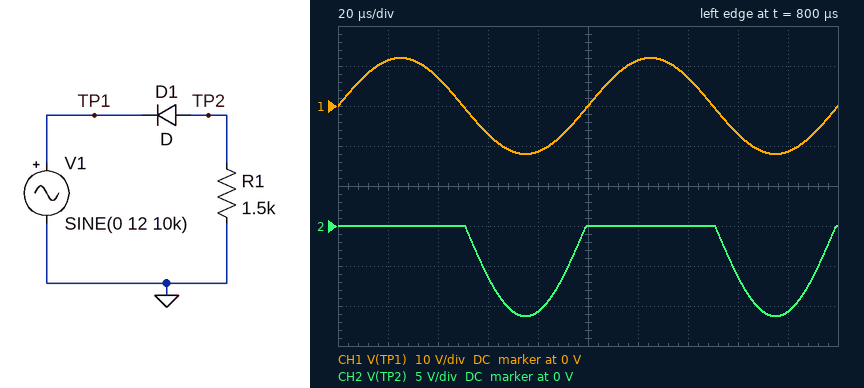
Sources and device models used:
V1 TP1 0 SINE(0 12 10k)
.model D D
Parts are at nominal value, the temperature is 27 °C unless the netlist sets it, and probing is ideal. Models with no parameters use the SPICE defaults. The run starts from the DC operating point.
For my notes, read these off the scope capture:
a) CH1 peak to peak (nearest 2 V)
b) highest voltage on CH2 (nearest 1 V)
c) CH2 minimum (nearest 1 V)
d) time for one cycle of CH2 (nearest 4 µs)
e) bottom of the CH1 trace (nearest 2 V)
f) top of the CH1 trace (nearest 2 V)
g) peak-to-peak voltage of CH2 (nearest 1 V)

24 V
0 V
-11 V
100 µs
-12 V
12 V
11 V
